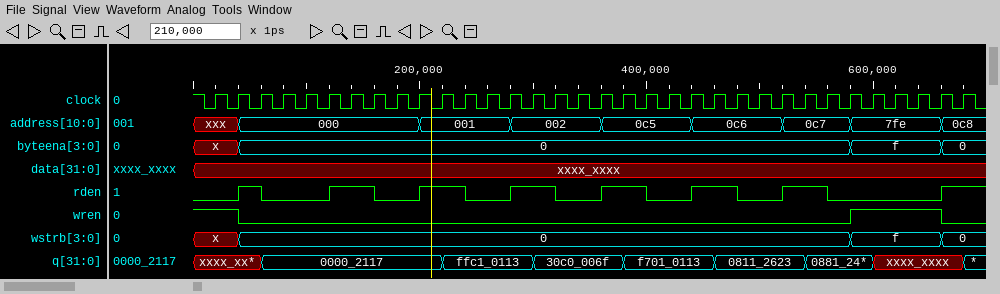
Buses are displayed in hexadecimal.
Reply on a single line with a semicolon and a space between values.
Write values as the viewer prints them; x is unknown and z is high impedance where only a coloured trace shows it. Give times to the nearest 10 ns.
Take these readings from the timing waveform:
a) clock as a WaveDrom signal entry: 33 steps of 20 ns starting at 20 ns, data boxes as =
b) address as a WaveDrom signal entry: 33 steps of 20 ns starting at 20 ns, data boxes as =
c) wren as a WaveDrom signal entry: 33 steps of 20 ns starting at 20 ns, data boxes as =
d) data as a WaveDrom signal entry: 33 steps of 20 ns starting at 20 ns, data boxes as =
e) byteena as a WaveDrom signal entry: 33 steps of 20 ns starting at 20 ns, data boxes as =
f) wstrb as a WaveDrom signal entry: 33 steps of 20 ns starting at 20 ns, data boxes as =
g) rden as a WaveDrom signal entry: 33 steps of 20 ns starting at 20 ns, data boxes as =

{name: 'clock', wave: 'p................................'}; {name: 'address', wave: 'x=.......=...=...=...=...=..=...=', data: '000 001 002 0c5 0c6 0c7 7fe 0c8'}; {name: 'wren', wave: '10..........................1...0'}; {name: 'data', wave: 'x................................'}; {name: 'byteena', wave: 'x=..........................=...=', data: '0 f 0'}; {name: 'wstrb', wave: 'x=..........................=...=', data: '0 f 0'}; {name: 'rden', wave: '010..1.0.1.0.1.0.1.0.1.0.1.0....1'}
